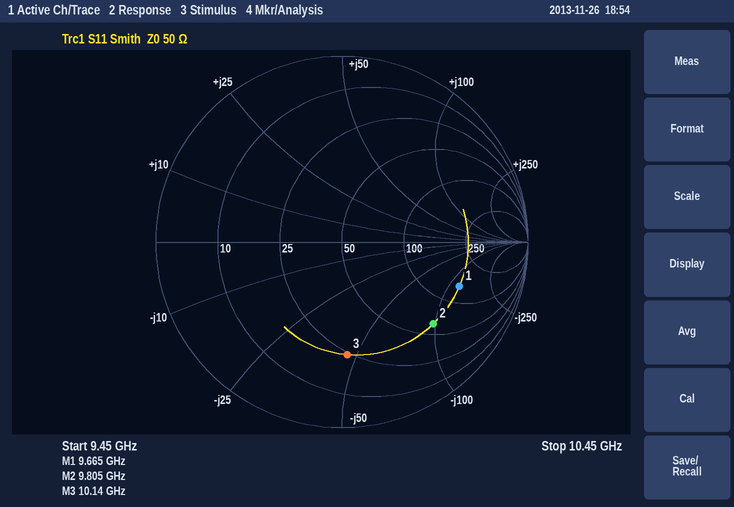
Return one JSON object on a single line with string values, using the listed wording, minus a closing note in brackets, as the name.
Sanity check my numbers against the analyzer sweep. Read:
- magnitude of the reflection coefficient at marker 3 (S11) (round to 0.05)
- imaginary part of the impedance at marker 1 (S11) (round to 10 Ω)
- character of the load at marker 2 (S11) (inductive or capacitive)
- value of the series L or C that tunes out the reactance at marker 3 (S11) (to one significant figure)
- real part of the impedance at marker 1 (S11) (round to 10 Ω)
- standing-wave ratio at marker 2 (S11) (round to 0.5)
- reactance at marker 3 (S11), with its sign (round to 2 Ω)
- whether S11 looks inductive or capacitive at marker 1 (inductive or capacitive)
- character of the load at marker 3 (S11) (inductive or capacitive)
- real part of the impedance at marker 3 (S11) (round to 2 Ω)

{"magnitude of the reflection coefficient at marker 3 (S11)": "0.60", "imaginary part of the impedance at marker 1 (S11)": "-120 Ω", "character of the load at marker 2 (S11)": "capacitive", "value of the series L or C that tunes out the reactance at marker 3 (S11)": "700 pH", "real part of the impedance at marker 1 (S11)": "140 Ω", "standing-wave ratio at marker 2 (S11)": "5.0", "reactance at marker 3 (S11), with its sign": "-46 Ω", "whether S11 looks inductive or capacitive at marker 1": "capacitive", "character of the load at marker 3 (S11)": "capacitive", "real part of the impedance at marker 3 (S11)": "24 Ω"}
